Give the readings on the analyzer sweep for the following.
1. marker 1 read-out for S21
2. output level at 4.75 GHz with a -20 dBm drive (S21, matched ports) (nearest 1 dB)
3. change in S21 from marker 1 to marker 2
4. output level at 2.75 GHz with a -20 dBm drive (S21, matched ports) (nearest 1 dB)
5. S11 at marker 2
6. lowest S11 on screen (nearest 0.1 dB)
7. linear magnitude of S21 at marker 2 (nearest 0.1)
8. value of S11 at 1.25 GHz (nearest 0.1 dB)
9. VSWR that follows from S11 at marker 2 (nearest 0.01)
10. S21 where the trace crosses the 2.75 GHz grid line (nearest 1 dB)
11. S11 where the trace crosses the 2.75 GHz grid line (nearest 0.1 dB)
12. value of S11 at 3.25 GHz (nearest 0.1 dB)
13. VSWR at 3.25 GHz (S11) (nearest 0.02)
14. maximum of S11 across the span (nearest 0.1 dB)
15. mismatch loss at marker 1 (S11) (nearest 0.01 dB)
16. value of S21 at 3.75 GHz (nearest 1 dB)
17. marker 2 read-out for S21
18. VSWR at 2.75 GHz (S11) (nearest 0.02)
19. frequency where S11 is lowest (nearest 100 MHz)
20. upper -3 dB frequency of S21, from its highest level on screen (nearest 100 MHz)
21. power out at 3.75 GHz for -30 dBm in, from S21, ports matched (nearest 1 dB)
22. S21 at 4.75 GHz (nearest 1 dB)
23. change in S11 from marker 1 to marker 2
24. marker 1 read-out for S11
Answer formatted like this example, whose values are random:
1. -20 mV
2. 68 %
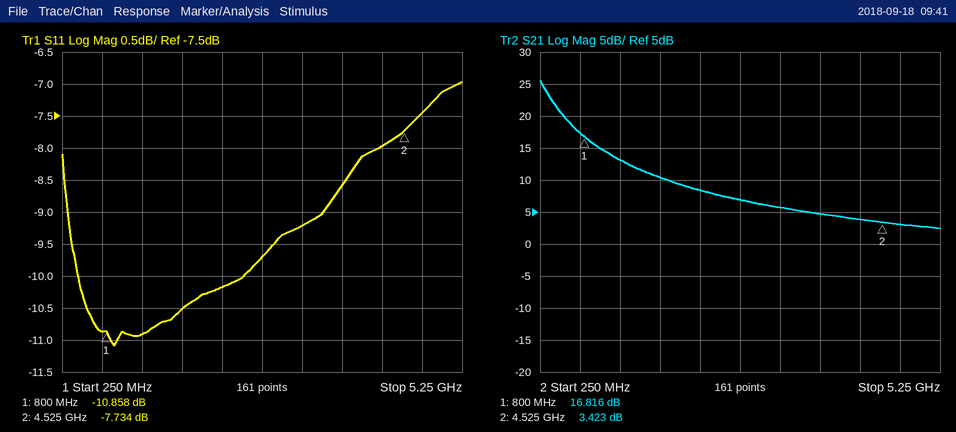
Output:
1. 16.816 dB
2. -17 dBm
3. -13.393 dB
4. -13 dBm
5. -7.734 dB
6. -11.1 dB
7. 1.5
8. -10.9 dB
9. 2.39
10. 7 dB
11. -9.7 dB
12. -9.2 dB
13. 2.06
14. -7.0 dB
15. 0.37 dB
16. 5 dB
17. 3.423 dB
18. 1.98
19. 900 MHz
20. 400 MHz
21. -25 dBm
22. 3 dB
23. 3.124 dB
24. -10.858 dB
